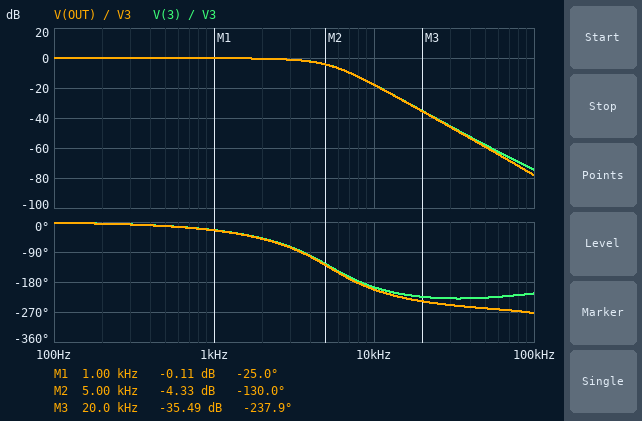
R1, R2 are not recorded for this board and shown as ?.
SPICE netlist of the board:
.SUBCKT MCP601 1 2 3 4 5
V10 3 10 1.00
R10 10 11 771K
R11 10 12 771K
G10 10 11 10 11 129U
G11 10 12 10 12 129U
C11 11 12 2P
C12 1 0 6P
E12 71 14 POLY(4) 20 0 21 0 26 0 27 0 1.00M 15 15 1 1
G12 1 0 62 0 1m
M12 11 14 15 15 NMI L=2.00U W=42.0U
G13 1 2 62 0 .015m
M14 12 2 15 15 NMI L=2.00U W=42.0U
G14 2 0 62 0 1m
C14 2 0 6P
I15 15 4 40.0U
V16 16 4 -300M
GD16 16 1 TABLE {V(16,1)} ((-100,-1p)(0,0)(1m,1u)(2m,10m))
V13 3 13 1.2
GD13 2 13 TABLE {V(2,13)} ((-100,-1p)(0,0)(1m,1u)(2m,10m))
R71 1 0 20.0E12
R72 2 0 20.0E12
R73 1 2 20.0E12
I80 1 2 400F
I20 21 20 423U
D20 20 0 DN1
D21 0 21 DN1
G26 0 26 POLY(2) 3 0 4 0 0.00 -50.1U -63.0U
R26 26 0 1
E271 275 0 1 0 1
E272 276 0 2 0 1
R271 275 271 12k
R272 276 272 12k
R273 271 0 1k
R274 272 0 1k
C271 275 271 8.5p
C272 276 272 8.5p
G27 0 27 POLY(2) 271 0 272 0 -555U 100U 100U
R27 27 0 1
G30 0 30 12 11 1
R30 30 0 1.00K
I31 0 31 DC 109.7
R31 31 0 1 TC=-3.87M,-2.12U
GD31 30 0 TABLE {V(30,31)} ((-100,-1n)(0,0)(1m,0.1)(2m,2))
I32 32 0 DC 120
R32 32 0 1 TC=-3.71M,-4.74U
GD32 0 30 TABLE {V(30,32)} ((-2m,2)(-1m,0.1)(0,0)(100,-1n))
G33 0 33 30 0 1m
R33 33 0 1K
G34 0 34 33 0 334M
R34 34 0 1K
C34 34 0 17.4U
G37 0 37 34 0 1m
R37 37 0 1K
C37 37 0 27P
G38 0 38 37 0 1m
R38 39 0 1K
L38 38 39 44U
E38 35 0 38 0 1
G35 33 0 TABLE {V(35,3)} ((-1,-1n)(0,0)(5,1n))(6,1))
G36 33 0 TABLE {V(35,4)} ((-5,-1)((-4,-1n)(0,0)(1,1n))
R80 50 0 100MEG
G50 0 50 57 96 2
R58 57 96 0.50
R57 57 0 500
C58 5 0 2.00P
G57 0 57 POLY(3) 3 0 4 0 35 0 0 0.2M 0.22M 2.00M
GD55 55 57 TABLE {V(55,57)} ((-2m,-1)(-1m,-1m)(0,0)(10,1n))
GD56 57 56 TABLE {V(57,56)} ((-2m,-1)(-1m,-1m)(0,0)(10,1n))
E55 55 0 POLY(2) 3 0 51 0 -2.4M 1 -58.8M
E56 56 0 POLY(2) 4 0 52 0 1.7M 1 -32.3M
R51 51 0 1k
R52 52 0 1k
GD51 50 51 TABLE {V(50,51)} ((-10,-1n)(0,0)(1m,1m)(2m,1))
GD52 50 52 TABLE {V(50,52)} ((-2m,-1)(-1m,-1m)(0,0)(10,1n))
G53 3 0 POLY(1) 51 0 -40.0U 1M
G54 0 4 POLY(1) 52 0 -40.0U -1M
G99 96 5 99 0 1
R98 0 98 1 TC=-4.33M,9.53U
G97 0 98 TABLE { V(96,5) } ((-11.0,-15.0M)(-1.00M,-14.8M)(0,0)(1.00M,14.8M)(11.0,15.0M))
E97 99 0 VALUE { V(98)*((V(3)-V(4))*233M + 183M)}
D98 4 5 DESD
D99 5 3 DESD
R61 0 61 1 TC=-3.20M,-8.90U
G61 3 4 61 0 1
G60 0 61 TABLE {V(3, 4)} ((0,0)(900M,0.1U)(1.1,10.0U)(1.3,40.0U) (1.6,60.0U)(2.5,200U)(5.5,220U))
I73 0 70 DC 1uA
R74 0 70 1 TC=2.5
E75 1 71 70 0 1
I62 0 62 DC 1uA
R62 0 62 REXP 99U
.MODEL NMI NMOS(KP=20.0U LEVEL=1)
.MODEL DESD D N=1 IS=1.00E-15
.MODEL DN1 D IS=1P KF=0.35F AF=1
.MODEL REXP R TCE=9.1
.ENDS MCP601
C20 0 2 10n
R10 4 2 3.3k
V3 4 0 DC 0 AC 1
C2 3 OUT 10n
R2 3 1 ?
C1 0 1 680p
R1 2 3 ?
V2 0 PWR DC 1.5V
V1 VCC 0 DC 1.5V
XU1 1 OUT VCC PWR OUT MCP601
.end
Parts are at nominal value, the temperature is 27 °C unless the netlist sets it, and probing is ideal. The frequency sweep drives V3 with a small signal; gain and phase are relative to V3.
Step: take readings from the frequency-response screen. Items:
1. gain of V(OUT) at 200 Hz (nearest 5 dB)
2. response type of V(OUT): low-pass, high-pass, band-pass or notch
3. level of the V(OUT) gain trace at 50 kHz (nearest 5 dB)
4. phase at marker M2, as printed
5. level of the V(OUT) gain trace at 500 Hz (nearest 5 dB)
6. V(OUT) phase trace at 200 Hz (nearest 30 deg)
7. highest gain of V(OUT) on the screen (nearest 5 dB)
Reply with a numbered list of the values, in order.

1. 0 dB
2. low-pass
3. -60 dB
4. -130.0 deg
5. 0 dB
6. 0 deg
7. 0 dB
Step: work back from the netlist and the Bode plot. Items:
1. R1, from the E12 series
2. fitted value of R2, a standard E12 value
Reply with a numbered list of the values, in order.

1. 47 kΩ
2. 2.7 kΩ
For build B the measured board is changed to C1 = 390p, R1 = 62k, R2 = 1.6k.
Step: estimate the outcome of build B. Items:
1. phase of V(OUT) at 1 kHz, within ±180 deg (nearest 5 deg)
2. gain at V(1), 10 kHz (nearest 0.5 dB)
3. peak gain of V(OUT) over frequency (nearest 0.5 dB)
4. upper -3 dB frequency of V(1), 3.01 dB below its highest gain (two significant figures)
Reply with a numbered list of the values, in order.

1. -20 deg
2. -12.0 dB
3. 0 dB
4. 4.8 kHz
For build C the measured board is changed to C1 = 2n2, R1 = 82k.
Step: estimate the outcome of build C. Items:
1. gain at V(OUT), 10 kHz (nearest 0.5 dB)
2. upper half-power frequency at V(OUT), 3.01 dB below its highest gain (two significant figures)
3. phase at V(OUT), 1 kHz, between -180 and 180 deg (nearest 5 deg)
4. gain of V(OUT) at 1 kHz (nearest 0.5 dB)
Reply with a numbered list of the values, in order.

1. -34.0 dB
2. 910 Hz
3. -70 deg
4. -3.5 dB
